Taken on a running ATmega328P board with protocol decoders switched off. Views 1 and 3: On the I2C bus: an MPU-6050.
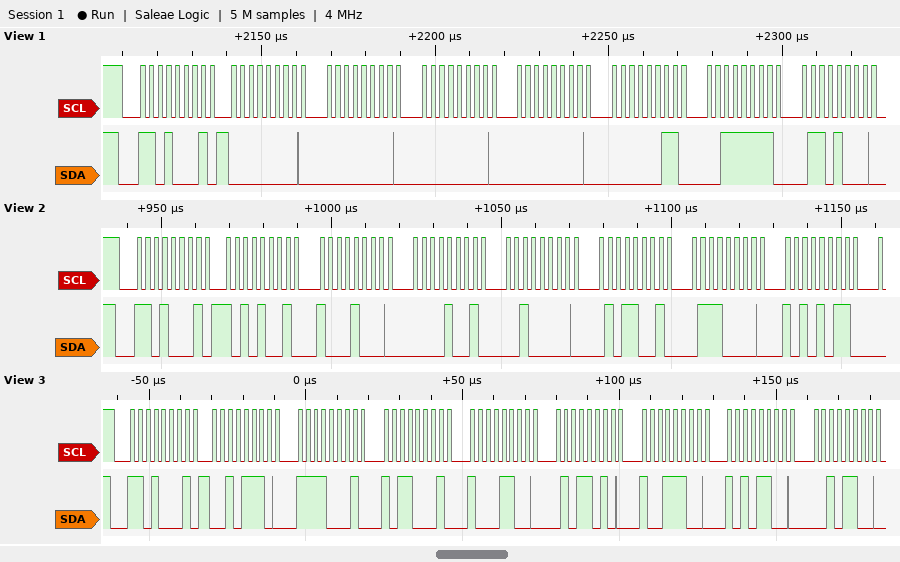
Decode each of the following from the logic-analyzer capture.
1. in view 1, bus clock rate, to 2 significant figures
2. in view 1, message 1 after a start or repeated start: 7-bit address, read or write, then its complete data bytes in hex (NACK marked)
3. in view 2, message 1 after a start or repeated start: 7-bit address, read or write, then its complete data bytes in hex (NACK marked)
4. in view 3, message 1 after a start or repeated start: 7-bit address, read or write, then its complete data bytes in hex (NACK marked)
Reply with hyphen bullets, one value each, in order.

- 400 kHz
- 0x68 read: 00 00 00 00 03 3F 68
- 0x68 read: A9 88 09 20 59 70 AB
- 0x68 read: 2E F1 B1 8C 5A 9C AC 2C
